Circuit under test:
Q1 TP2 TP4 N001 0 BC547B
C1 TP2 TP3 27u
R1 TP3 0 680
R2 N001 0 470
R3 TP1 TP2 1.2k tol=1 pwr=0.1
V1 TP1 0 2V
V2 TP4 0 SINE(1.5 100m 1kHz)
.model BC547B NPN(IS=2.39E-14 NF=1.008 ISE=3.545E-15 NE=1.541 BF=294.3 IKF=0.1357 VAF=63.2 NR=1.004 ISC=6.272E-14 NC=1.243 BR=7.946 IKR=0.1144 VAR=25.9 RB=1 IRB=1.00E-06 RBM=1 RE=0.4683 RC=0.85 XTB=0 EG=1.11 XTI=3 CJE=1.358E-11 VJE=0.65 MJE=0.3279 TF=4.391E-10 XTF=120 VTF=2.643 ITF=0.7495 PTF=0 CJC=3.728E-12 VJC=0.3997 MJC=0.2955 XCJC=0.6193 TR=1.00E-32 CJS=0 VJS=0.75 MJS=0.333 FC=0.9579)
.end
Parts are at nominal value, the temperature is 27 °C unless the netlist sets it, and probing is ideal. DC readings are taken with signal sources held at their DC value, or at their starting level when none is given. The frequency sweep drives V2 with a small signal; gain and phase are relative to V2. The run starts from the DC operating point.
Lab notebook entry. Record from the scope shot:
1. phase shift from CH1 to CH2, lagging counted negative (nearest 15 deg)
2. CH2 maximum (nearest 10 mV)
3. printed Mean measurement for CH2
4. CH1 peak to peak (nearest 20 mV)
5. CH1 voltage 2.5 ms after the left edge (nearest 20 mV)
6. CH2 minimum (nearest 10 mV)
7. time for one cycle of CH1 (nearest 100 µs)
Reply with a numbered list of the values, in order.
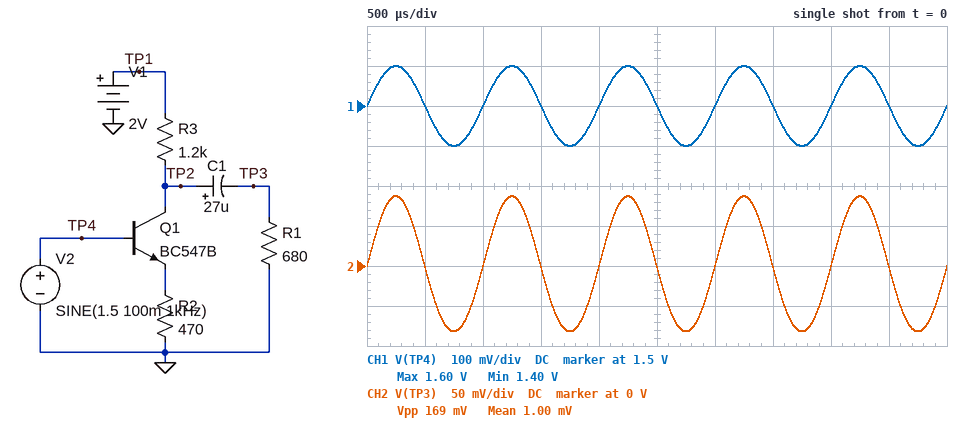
1. 0 deg
2. 90 mV
3. 1.00 mV
4. 200 mV
5. 1.50 V
6. -80 mV
7. 1.0 ms
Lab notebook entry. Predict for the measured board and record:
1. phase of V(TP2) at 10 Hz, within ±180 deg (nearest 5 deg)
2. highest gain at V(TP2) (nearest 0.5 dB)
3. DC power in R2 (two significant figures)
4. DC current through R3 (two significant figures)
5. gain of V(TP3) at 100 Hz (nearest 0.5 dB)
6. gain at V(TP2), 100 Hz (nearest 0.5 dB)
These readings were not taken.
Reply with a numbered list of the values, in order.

1. 0 deg
2. -1.0 dB
3. 1.4 mW
4. 980 µA
5. -1.5 dB
6. -1.5 dB
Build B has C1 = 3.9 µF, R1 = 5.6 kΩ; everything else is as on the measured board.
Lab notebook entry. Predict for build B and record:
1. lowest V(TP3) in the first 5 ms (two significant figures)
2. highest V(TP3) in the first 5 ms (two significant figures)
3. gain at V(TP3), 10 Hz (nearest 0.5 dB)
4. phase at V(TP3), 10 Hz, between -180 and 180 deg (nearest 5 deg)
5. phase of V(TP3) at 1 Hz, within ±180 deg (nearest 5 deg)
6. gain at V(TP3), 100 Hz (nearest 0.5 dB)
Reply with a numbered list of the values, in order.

1. -88 mV
2. 90 mV
3. -3.0 dB
4. 35 deg
5. 80 deg
6. -1.0 dB
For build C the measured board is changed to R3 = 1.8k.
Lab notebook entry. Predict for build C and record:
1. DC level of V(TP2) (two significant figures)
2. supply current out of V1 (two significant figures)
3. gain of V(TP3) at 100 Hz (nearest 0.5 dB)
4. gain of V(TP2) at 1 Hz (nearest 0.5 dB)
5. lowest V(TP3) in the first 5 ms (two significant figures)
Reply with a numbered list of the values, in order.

1. 810 mV
2. 660 µA
3. -1.0 dB
4. -0.5 dB
5. -89 mV
